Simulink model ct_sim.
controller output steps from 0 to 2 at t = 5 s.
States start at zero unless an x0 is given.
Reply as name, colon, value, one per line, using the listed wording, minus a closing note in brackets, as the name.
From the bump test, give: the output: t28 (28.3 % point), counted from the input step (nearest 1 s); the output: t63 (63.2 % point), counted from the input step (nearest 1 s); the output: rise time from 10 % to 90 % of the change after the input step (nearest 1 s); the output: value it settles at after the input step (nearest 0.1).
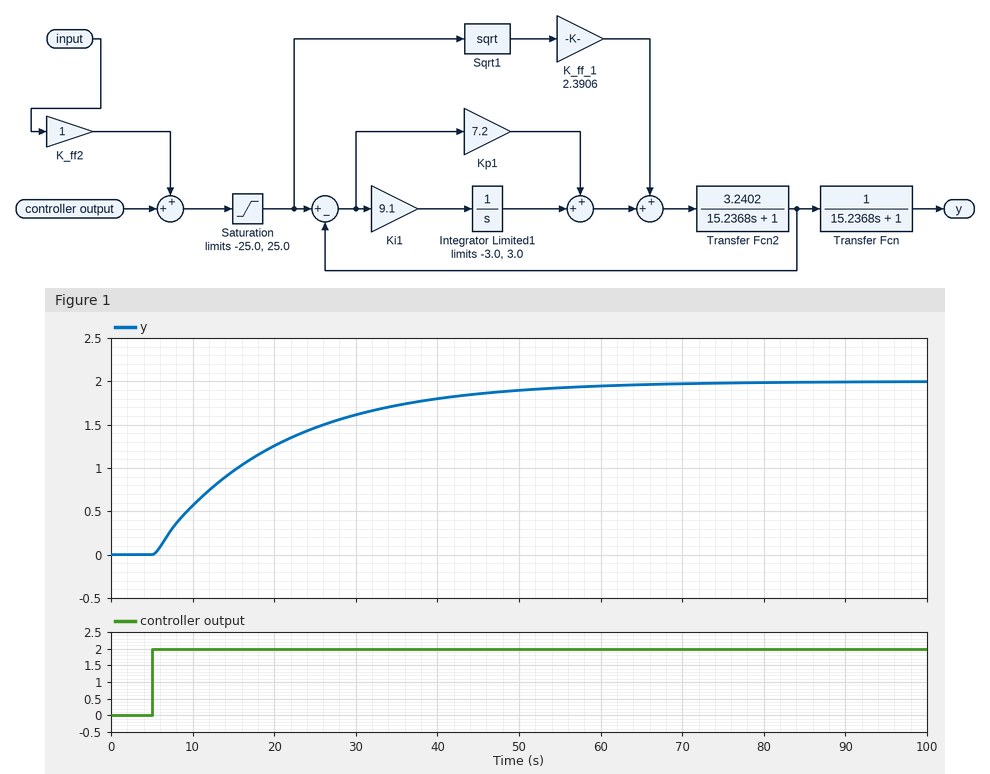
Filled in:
the output: t28 (28.3 % point), counted from the input step: 5 s
the output: t63 (63.2 % point), counted from the input step: 15 s
the output: rise time from 10 % to 90 % of the change after the input step: 33 s
the output: value it settles at after the input step: 2.0
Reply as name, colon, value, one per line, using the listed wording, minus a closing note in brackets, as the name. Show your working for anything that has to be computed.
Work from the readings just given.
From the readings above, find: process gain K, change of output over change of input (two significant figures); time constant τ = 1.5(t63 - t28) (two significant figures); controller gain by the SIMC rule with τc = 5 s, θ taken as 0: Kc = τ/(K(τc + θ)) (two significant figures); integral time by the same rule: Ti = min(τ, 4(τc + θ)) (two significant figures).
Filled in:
process gain K, change of output over change of input: (2 - 0) / 2 = 1.0
time constant τ = 1.5(t63 - t28): 1.5 × (15 - 5) = 15 s
controller gain by the SIMC rule with τc = 5 s, θ taken as 0: Kc = τ/(K(τc + θ)): 15 / (1 × (5 + 0)) = 3.0
integral time by the same rule: Ti = min(τ, 4(τc + θ)): min(15, 4 × (5 + 0)) = 15 s
